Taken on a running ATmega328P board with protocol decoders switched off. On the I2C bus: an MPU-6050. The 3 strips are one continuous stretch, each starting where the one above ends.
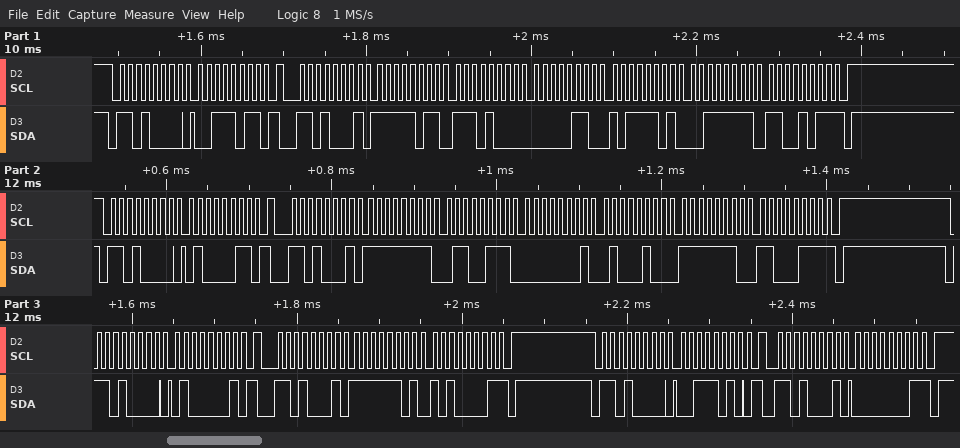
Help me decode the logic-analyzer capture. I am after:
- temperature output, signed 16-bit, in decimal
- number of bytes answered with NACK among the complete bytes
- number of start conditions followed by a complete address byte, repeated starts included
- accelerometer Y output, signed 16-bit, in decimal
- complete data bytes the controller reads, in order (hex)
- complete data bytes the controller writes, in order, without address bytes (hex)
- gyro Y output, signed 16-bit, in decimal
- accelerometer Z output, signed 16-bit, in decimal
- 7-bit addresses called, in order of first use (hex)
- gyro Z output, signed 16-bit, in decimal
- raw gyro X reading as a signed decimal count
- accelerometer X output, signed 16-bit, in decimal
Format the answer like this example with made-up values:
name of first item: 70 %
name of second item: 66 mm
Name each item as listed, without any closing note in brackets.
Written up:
temperature output, signed 16-bit, in decimal: -607
number of bytes answered with NACK among the complete bytes: 4
number of start conditions followed by a complete address byte, repeated starts included: 8
accelerometer Y output, signed 16-bit, in decimal: 1725
complete data bytes the controller reads, in order: FB E8 06 BD 3F CB FF 67 01 44 FE C7 FD A1 01
complete data bytes the controller writes, in order, without address bytes: 3B 43 41 3A
gyro Y output, signed 16-bit, in decimal: 324
accelerometer Z output, signed 16-bit, in decimal: 16331
7-bit addresses called, in order of first use: 0x68
gyro Z output, signed 16-bit, in decimal: -313
raw gyro X reading as a signed decimal count: -153
accelerometer X output, signed 16-bit, in decimal: -1048
